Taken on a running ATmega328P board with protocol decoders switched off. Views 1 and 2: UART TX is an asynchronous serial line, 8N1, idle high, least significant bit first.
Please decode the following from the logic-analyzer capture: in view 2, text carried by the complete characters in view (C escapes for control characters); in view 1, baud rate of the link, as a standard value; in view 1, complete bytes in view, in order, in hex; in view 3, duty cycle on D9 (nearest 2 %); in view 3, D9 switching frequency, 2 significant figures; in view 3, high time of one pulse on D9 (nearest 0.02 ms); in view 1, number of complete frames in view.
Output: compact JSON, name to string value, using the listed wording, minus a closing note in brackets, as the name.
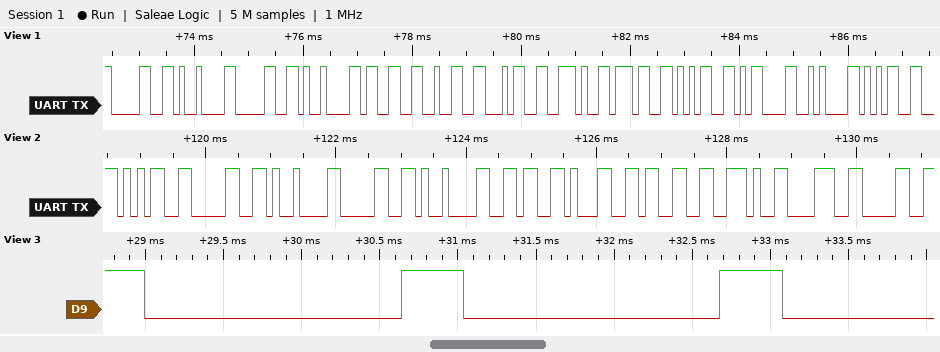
{"in view 2, text carried by the complete characters in view": "\"50\\t0\\t613.80\"", "in view 1, baud rate of the link, as a standard value": "9600 baud", "in view 1, complete bytes in view, in order, in hex": "30 09 30 09 33 32 34 2E 37 35 0D 0A 35", "in view 3, duty cycle on D9": "20 %", "in view 3, D9 switching frequency, 2 significant figures": "490 Hz", "in view 3, high time of one pulse on D9": "0.40 ms", "in view 1, number of complete frames in view": "13"}
